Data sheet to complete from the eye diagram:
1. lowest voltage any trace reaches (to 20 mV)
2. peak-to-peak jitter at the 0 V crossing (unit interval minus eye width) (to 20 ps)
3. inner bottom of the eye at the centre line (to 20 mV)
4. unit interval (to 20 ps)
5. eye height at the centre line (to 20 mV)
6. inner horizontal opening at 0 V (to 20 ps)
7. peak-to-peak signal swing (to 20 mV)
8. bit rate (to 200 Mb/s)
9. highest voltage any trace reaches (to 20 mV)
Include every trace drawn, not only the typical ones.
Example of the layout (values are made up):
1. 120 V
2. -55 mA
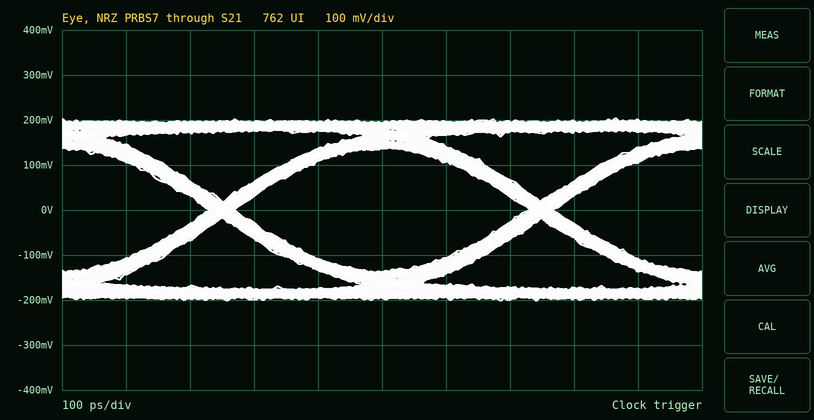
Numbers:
1. -200 mV
2. 40 ps
3. -140 mV
4. 500 ps
5. 280 mV
6. 460 ps
7. 400 mV
8. 2.0 Gb/s
9. 200 mV
